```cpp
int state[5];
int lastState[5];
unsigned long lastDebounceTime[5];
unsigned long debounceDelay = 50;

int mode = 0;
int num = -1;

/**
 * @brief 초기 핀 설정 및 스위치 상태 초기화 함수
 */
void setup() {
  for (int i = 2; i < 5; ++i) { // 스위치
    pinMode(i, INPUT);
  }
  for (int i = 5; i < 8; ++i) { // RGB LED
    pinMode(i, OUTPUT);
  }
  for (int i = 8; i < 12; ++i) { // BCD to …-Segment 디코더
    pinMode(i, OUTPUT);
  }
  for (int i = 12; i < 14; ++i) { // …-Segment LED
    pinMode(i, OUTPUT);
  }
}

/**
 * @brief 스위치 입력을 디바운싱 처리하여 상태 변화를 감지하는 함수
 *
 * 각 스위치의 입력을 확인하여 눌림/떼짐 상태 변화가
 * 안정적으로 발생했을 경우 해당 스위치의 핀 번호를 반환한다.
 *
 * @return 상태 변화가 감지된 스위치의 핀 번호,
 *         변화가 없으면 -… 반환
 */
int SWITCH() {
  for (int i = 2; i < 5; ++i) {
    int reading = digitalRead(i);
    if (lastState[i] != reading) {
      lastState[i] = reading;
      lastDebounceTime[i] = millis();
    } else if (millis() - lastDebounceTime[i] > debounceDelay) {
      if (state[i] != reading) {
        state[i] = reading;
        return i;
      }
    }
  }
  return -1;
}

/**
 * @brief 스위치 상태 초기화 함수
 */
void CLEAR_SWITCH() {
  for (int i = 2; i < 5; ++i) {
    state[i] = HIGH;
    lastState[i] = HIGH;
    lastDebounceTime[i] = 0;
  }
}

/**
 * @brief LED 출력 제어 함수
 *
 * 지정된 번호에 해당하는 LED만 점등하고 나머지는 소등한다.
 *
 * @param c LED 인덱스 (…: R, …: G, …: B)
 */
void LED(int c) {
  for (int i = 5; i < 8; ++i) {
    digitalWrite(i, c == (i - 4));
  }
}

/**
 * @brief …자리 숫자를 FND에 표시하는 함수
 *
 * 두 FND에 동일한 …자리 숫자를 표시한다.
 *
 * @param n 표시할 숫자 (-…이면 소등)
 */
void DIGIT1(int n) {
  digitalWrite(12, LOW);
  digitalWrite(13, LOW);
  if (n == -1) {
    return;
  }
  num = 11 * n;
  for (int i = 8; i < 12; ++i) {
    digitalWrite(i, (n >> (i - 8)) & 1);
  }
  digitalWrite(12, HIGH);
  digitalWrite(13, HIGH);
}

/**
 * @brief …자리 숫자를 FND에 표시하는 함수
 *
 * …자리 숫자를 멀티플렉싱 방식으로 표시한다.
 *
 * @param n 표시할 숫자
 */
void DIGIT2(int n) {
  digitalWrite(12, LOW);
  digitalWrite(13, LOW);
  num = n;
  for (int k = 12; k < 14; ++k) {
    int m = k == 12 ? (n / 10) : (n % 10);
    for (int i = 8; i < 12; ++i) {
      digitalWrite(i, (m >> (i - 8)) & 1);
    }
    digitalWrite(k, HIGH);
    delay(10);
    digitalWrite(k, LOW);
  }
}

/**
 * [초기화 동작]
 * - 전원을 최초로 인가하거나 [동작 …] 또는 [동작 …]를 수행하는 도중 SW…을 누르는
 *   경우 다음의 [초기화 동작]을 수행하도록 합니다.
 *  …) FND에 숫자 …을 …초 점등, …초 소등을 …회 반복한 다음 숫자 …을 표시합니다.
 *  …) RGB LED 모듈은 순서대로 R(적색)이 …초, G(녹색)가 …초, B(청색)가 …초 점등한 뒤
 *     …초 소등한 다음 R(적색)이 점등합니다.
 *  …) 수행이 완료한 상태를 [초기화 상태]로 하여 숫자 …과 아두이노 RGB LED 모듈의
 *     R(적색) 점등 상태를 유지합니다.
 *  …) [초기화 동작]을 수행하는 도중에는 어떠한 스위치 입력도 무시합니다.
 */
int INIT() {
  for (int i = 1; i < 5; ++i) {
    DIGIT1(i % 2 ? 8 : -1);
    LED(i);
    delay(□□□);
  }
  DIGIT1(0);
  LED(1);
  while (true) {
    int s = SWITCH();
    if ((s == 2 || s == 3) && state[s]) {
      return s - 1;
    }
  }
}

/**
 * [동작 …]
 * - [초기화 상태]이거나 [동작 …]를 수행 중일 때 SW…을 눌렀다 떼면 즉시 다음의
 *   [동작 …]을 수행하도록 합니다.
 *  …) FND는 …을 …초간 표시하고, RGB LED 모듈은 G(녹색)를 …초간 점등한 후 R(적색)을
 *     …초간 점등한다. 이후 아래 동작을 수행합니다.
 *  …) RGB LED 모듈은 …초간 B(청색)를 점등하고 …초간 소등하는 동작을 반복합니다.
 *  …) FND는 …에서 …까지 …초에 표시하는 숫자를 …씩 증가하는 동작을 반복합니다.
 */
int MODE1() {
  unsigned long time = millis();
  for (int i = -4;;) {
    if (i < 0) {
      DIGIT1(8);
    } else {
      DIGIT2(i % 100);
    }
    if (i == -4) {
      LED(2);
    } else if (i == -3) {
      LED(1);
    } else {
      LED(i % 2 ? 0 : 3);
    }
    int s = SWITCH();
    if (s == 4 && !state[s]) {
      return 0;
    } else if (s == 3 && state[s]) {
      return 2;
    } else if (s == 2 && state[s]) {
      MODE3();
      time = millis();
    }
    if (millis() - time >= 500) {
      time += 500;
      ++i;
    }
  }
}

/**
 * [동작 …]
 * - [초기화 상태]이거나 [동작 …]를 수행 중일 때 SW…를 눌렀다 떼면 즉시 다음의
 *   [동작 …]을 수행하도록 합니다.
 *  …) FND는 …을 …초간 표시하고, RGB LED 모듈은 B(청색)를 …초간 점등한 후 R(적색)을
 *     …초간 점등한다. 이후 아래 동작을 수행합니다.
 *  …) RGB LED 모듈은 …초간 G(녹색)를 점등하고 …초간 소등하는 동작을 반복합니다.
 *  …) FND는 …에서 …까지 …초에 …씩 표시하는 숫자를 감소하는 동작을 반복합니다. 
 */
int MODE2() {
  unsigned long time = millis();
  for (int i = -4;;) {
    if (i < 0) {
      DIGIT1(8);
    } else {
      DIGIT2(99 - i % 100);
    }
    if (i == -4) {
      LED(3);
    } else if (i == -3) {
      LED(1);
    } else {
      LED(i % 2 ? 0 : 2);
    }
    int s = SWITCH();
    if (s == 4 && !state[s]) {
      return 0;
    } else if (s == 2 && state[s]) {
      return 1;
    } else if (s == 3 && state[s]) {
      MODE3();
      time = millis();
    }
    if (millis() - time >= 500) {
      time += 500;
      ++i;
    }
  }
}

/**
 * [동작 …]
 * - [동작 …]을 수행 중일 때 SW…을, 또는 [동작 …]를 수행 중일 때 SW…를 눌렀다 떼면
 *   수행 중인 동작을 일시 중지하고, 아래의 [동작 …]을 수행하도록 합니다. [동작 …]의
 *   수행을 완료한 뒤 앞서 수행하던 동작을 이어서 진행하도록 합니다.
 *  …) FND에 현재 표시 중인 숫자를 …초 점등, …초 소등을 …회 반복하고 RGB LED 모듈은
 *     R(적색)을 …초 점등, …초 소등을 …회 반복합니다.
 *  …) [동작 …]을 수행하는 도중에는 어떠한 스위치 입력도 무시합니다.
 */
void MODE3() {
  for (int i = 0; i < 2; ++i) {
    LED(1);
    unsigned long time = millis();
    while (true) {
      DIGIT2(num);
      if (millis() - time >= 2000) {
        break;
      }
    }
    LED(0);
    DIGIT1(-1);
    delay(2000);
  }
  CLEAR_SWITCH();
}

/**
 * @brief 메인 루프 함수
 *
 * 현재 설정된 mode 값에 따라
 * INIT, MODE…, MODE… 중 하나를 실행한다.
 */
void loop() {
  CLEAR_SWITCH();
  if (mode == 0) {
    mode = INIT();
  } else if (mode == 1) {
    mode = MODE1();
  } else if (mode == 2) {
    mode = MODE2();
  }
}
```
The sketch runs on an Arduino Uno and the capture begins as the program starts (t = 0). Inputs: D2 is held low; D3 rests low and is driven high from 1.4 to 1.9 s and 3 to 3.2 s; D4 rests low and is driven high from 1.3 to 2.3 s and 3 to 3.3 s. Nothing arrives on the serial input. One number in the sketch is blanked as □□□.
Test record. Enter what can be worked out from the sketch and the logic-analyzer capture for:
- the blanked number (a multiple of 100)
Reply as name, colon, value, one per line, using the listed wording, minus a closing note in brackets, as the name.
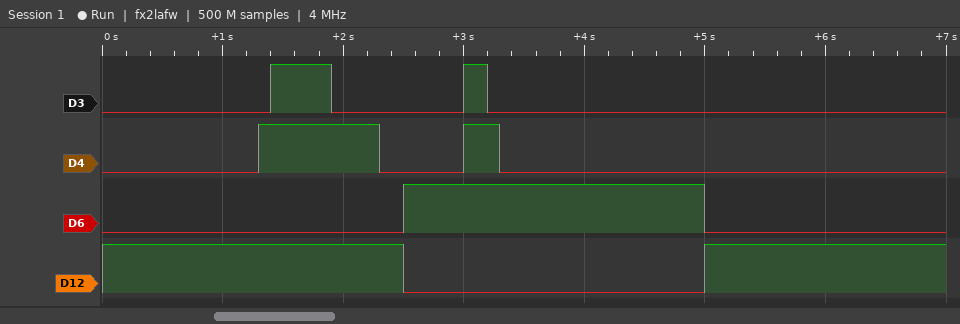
the blanked number: 2500
